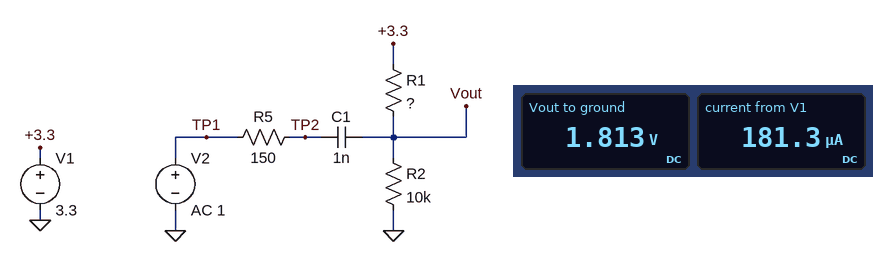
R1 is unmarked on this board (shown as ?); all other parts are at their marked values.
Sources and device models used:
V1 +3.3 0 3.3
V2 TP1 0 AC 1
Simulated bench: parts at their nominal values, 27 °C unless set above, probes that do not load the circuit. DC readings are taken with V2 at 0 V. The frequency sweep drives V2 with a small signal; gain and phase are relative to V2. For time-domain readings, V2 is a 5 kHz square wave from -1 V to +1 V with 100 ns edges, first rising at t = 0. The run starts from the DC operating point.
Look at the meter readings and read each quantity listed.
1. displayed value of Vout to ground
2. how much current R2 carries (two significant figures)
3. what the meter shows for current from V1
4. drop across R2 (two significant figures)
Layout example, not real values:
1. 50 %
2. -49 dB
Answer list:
1. 1.813 V
2. 180 µA
3. 181.3 µA
4. 1.8 V
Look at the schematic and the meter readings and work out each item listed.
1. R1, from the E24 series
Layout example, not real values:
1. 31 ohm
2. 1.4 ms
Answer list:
1. 8.2 kΩ
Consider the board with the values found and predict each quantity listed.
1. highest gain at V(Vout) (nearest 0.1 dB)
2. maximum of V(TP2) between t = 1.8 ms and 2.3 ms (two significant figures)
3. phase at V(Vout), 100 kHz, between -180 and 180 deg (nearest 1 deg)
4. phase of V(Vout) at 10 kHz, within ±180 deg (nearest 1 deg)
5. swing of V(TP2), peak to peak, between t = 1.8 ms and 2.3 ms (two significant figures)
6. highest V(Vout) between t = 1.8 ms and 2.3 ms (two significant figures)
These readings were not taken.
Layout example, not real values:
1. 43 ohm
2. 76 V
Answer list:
1. -0.3 dB
2. 1.0 V
3. 19 deg
4. 74 deg
5. 2.0 V
6. 3.7 V
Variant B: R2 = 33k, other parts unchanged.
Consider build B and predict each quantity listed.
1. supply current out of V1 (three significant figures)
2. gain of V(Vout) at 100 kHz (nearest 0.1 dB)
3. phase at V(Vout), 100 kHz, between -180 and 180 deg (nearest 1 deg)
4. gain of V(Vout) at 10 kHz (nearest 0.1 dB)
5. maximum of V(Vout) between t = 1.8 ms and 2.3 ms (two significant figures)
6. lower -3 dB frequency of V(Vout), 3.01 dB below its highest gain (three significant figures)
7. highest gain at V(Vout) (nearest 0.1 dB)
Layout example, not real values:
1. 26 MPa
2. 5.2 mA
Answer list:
1. 80.1 µA
2. -0.4 dB
3. 13 deg
4. -8.4 dB
5. 4.6 V
6. 23.7 kHz
7. -0.2 dB
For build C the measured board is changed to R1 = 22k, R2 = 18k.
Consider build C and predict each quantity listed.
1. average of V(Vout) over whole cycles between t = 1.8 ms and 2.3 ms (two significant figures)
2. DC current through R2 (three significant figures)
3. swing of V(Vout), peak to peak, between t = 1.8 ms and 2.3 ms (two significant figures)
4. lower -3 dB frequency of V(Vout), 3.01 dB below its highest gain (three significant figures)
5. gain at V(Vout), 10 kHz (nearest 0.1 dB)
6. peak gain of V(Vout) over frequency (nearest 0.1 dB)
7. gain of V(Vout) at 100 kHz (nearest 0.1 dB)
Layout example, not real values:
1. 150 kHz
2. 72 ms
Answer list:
1. 1.5 V
2. 82.5 µA
3. 3.9 V
4. 15.8 kHz
5. -5.6 dB
6. -0.1 dB
7. -0.2 dB
